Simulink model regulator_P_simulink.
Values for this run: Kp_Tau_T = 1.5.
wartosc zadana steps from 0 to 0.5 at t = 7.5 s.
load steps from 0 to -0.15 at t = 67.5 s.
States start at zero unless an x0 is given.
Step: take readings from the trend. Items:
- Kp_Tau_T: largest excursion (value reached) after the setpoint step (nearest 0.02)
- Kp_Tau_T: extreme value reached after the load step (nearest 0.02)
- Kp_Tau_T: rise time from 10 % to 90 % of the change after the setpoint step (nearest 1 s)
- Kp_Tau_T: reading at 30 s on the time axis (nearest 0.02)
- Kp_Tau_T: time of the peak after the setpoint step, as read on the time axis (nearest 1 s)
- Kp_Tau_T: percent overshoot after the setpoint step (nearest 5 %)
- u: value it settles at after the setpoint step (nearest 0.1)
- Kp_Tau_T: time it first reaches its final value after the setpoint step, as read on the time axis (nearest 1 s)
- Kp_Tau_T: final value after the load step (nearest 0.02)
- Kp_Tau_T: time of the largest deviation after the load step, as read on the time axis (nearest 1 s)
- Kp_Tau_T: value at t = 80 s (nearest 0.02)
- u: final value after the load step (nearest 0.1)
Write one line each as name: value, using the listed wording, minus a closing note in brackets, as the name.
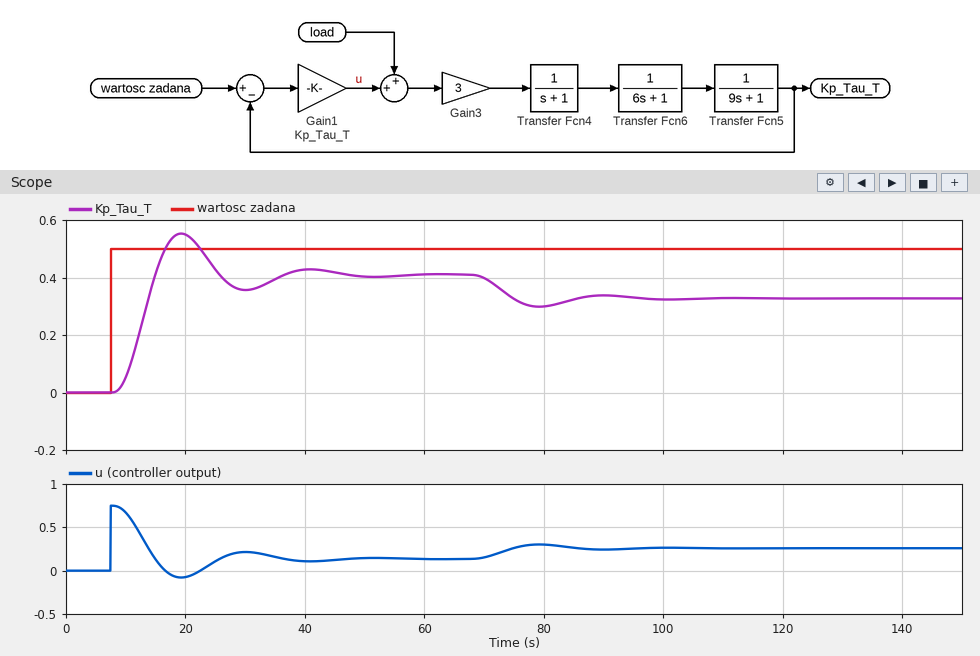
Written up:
Kp_Tau_T: largest excursion (value reached) after the setpoint step: 0.56
Kp_Tau_T: extreme value reached after the load step: 0.30
Kp_Tau_T: rise time from 10 % to 90 % of the change after the setpoint step: 5 s
Kp_Tau_T: reading at 30 s on the time axis: 0.36
Kp_Tau_T: time of the peak after the setpoint step, as read on the time axis: 19 s
Kp_Tau_T: percent overshoot after the setpoint step: 35 %
u: value it settles at after the setpoint step: 0.1
Kp_Tau_T: time it first reaches its final value after the setpoint step, as read on the time axis: 15 s
Kp_Tau_T: final value after the load step: 0.32
Kp_Tau_T: time of the largest deviation after the load step, as read on the time axis: 79 s
Kp_Tau_T: value at t = 80 s: 0.30
u: final value after the load step: 0.3
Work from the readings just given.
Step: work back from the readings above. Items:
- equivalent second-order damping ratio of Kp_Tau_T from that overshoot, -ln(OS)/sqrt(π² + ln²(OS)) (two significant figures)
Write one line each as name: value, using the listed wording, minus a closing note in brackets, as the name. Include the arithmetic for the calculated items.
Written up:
equivalent second-order damping ratio of Kp_Tau_T from that overshoot, -ln(OS)/sqrt(π² + ln²(OS)): ln(0.35) = -1.050; 1.050 / sqrt(9.870 + 1.102) = 0.32
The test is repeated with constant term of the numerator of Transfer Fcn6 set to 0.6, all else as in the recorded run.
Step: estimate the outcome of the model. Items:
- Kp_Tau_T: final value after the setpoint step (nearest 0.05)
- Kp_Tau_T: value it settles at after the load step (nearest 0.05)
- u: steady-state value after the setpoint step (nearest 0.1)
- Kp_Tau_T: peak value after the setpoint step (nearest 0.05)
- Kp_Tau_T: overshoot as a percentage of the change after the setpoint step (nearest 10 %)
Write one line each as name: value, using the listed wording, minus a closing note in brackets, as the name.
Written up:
Kp_Tau_T: final value after the setpoint step: 0.35
Kp_Tau_T: value it settles at after the load step: 0.30
u: steady-state value after the setpoint step: 0.2
Kp_Tau_T: peak value after the setpoint step: 0.45
Kp_Tau_T: overshoot as a percentage of the change after the setpoint step: 20 %
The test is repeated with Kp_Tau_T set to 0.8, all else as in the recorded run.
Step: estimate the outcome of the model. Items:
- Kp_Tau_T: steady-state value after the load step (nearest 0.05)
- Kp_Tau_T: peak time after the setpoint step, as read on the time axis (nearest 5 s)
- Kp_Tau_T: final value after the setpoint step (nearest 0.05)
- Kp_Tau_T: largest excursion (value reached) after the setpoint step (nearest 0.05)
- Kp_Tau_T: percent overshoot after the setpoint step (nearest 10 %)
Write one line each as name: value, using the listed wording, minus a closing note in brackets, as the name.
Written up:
Kp_Tau_T: steady-state value after the load step: 0.20
Kp_Tau_T: peak time after the setpoint step, as read on the time axis: 25 s
Kp_Tau_T: final value after the setpoint step: 0.35
Kp_Tau_T: largest excursion (value reached) after the setpoint step: 0.40
Kp_Tau_T: percent overshoot after the setpoint step: 20 %
